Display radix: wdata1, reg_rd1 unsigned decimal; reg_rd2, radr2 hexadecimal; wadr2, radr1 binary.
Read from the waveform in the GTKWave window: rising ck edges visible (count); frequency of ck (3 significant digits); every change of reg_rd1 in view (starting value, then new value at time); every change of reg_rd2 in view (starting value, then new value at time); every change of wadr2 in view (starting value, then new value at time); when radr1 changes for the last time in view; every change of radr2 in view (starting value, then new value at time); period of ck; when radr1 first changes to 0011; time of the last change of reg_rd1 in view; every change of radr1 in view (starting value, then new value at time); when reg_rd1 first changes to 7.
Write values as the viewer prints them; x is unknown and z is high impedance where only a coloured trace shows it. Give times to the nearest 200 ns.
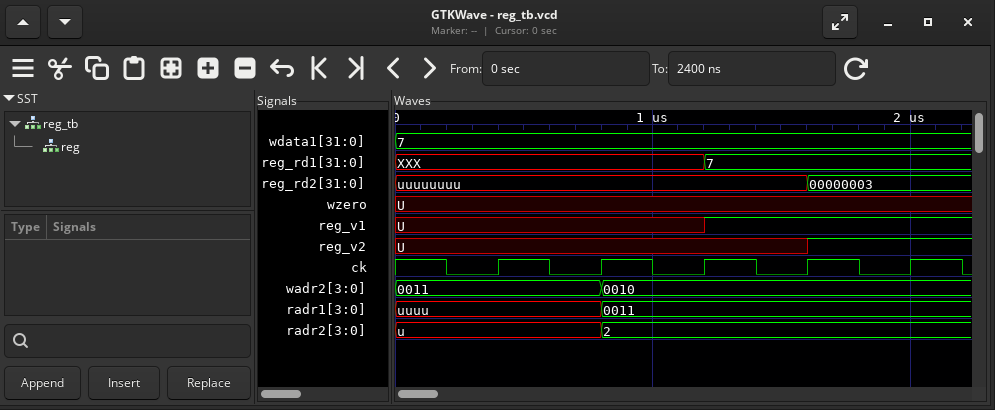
5
2.50 MHz
XXX, 7 at 1200 ns
uuuuuuuu, 00000003 at 1600 ns
0011, 0010 at 800 ns
800 ns
u, 2 at 800 ns
400 ns
800 ns
1200 ns
uuuu, 0011 at 800 ns
1200 ns
